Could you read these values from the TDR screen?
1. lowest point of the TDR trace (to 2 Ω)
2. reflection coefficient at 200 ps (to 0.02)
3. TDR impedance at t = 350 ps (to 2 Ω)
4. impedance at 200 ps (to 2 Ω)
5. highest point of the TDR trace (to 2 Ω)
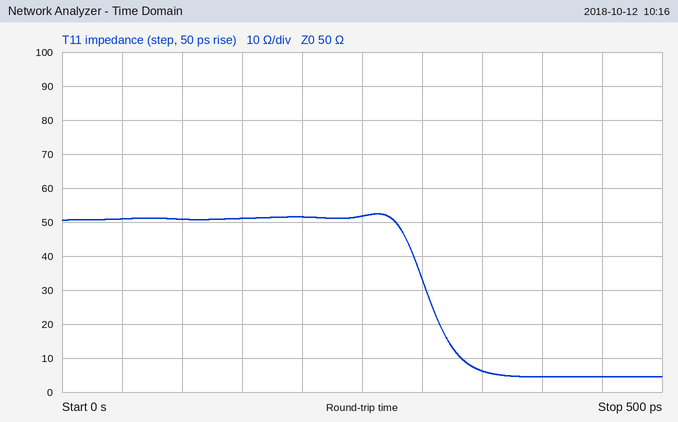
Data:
4 Ω
+0.02
6 Ω
52 Ω
52 Ω
